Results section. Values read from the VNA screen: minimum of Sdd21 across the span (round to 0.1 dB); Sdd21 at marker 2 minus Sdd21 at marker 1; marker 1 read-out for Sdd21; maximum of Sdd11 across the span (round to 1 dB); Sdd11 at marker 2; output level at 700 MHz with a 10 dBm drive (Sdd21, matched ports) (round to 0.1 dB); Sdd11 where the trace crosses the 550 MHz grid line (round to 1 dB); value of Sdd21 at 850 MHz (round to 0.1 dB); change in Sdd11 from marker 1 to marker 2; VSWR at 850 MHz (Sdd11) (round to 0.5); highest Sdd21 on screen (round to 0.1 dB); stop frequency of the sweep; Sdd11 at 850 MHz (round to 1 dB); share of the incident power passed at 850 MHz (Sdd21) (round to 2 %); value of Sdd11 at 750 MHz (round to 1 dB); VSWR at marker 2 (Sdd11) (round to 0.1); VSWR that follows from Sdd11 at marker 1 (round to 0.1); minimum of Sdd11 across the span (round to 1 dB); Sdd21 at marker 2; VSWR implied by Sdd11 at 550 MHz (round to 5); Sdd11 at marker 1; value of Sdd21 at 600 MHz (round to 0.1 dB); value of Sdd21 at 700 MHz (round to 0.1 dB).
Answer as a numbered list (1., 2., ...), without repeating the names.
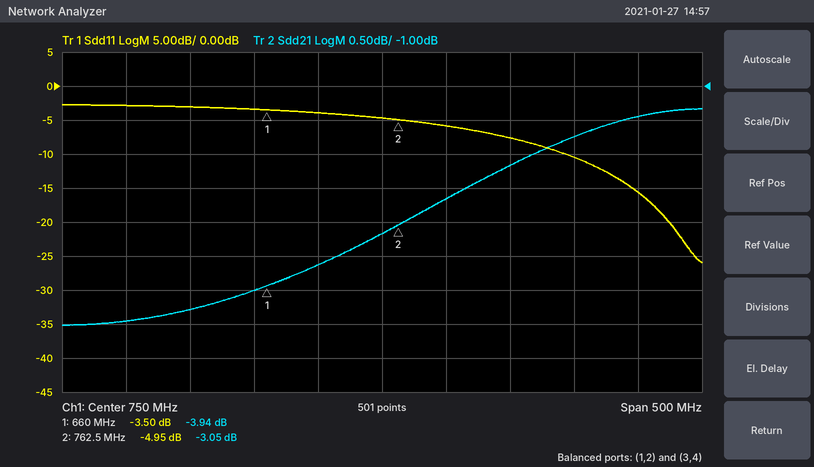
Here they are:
1. -4.5 dB
2. 0.89 dB
3. -3.94 dB
4. -3 dB
5. -4.95 dB
6. 6.4 dBm
7. -3 dB
8. -2.2 dB
9. -1.45 dB
10. 2.5
11. -1.3 dB
12. 1 GHz
13. -8 dB
14. 60 %
15. -5 dB
16. 3.6
17. 5.0
18. -26 dB
19. -3.05 dB
20. 5
21. -3.50 dB
22. -4.3 dB
23. -3.6 dB
